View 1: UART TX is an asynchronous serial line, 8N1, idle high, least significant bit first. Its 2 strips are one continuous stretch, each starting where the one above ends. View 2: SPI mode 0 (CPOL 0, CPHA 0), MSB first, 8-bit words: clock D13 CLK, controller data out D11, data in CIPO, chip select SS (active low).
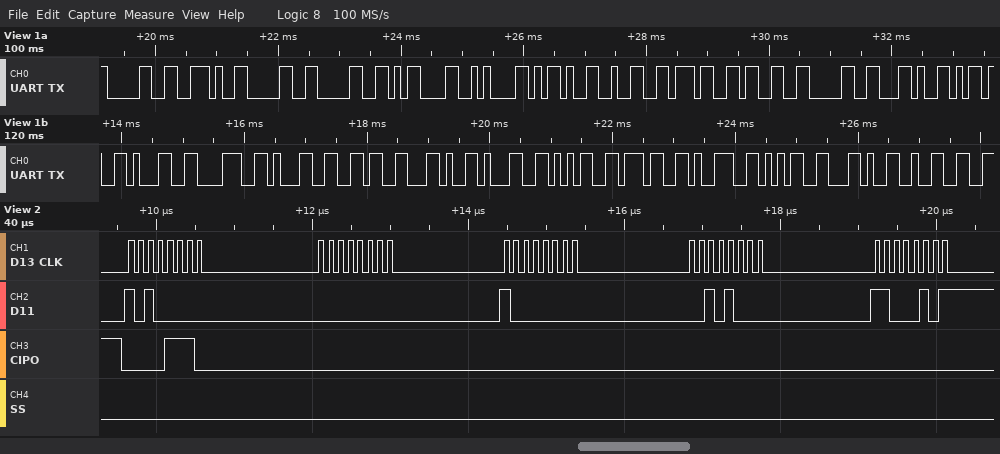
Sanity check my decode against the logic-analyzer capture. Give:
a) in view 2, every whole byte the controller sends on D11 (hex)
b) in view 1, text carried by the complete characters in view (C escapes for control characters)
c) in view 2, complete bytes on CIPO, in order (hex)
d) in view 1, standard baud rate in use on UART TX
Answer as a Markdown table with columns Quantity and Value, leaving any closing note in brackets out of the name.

| Quantity | Value |
|---|---|
| in view 2, every whole byte the controller sends on D11 | A0 00 80 28 C5 |
| in view 1, text carried by the complete characters in view | "0.00\r\n-2730,-1816,15795,2" |
| in view 2, complete bytes on CIPO, in order | 0E 00 00 00 00 |
| in view 1, standard baud rate in use on UART TX | 9600 baud |
